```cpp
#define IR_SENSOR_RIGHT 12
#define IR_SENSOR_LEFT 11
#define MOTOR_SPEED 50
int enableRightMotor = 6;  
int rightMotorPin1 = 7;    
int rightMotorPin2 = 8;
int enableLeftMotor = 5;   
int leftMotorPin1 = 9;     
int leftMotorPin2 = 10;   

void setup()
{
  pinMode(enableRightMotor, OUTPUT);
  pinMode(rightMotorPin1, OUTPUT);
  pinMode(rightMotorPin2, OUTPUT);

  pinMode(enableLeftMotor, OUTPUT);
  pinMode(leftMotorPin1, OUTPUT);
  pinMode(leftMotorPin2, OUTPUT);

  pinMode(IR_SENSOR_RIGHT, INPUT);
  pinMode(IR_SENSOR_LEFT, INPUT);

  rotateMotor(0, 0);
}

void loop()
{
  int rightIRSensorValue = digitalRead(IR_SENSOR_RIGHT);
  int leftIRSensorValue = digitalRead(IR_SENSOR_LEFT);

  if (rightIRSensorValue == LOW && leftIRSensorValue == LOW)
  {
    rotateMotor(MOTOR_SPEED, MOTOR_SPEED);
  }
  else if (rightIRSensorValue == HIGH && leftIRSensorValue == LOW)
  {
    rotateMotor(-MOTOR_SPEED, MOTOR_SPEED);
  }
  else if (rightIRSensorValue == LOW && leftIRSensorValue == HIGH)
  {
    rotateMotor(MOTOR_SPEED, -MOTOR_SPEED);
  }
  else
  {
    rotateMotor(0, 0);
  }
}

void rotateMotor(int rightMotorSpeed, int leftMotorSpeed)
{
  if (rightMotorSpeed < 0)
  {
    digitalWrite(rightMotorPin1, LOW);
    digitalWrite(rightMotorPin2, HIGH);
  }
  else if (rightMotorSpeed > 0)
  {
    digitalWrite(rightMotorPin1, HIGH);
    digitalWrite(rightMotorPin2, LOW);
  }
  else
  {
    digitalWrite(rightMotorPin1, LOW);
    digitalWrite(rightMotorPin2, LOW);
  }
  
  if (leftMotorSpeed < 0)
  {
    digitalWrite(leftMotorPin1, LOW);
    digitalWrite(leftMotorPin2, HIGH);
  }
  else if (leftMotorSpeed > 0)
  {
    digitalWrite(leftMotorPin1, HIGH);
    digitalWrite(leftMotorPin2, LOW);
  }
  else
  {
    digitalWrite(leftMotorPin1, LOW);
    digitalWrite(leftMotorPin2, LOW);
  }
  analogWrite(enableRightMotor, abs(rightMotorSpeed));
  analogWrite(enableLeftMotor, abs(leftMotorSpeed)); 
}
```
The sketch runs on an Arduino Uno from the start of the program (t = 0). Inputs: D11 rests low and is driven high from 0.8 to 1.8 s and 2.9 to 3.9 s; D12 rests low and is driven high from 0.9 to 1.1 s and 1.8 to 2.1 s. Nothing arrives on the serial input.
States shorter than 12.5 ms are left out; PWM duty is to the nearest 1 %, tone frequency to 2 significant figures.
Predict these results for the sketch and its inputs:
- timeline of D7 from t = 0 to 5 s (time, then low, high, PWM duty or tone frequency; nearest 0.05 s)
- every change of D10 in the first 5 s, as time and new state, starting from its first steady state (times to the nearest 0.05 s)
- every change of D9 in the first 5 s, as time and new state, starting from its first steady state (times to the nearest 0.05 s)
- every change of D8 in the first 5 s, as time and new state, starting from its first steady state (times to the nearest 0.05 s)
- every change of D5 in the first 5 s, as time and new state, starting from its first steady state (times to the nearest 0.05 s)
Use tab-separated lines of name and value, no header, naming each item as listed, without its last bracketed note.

timeline of D7 from t = 0 to 5 s	0 s high; 0.9 s low; 1.1 s high; 1.8 s low; 2.1 s high
every change of D10 in the first 5 s, as time and new state, starting from its first steady state	0 s low; 0.8 s high; 0.9 s low; 1.1 s high; 1.8 s low; 2.9 s high; 3.9 s low
every change of D9 in the first 5 s, as time and new state, starting from its first steady state	0 s high; 0.8 s low; 1.8 s high; 2.9 s low; 3.9 s high
every change of D8 in the first 5 s, as time and new state, starting from its first steady state	0 s low; 1.8 s high; 2.1 s low
every change of D5 in the first 5 s, as time and new state, starting from its first steady state	0 s PWM 20 %; 0.9 s low; 1.1 s PWM 20 %
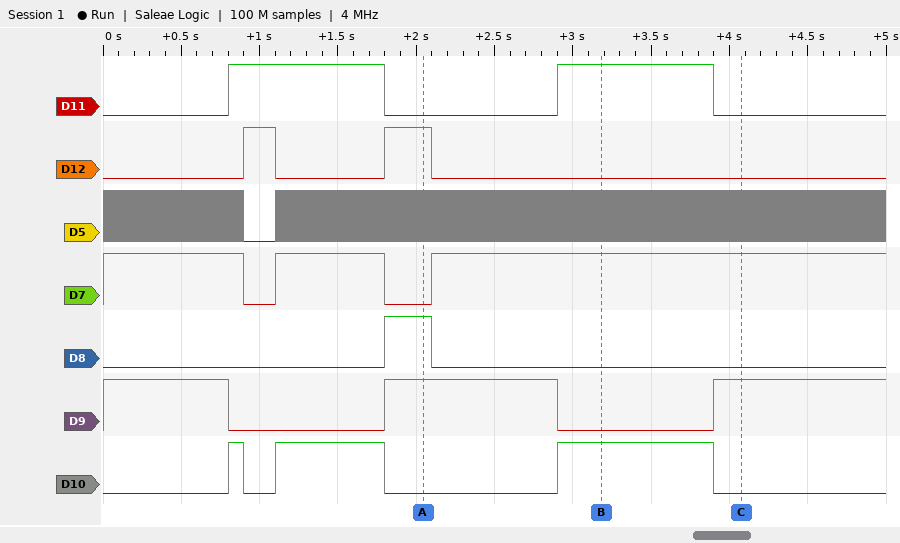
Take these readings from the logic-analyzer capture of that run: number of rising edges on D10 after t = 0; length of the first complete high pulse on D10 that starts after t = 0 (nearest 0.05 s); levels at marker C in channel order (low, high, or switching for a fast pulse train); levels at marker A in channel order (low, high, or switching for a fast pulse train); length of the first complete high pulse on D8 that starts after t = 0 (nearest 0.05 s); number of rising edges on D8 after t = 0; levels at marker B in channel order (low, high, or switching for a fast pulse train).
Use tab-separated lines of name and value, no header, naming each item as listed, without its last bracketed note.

number of rising edges on D10 after t = 0	3
length of the first complete high pulse on D10 that starts after t = 0	0.10 s
levels at marker C in channel order	D11 low, D12 low, D5 switching, D7 high, D8 low, D9 high, D10 low
levels at marker A in channel order	D11 low, D12 high, D5 switching, D7 low, D8 high, D9 high, D10 low
length of the first complete high pulse on D8 that starts after t = 0	0.30 s
number of rising edges on D8 after t = 0	1
levels at marker B in channel order	D11 high, D12 low, D5 switching, D7 high, D8 low, D9 low, D10 high
